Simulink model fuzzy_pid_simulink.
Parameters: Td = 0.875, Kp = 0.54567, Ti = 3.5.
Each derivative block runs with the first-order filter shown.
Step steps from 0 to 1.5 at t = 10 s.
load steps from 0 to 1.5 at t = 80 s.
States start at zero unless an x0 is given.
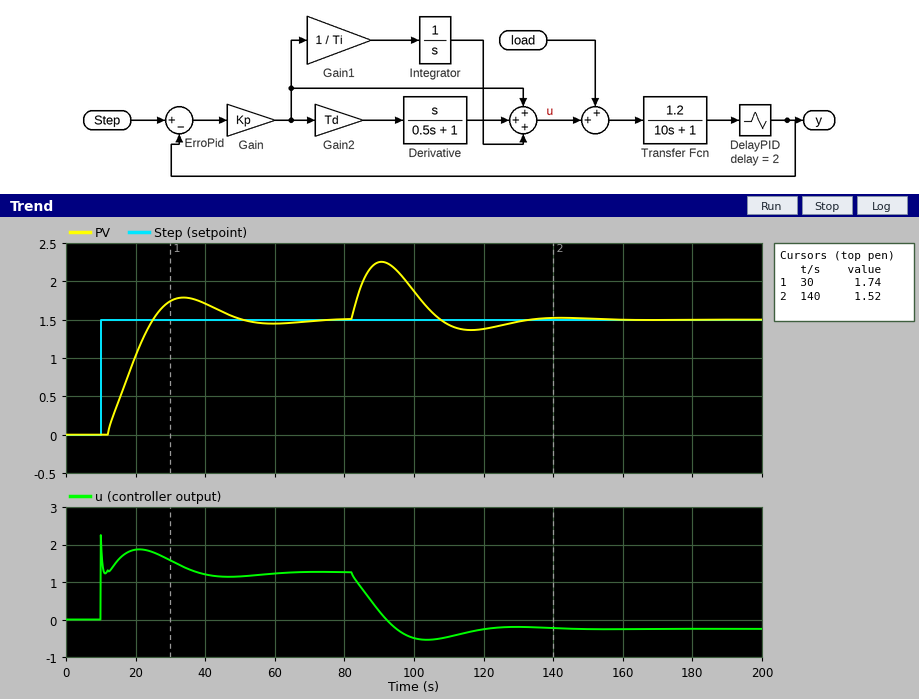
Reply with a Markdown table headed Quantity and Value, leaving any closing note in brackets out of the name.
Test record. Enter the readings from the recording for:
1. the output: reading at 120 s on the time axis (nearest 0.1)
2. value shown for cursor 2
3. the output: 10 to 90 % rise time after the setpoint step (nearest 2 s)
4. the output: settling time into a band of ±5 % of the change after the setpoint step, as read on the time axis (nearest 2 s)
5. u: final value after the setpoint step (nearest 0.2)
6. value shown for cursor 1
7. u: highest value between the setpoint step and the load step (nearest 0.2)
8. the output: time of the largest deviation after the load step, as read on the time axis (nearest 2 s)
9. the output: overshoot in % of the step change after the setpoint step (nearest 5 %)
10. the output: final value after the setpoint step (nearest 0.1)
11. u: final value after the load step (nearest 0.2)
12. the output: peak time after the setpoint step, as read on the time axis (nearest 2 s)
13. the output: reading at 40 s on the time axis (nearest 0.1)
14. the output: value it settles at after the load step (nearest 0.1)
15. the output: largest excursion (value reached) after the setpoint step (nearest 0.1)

| Quantity | Value |
|---|---|
| the output: reading at 120 s on the time axis | 1.4 |
| value shown for cursor 2 | 1.52 |
| the output: 10 to 90 % rise time after the setpoint step | 10 s |
| the output: settling time into a band of ±5 % of the change after the setpoint step, as read on the time axis | 46 s |
| u: final value after the setpoint step | 1.2 |
| value shown for cursor 1 | 1.74 |
| u: highest value between the setpoint step and the load step | 2.2 |
| the output: time of the largest deviation after the load step, as read on the time axis | 90 s |
| the output: overshoot in % of the step change after the setpoint step | 20 % |
| the output: final value after the setpoint step | 1.5 |
| u: final value after the load step | -0.2 |
| the output: peak time after the setpoint step, as read on the time axis | 34 s |
| the output: reading at 40 s on the time axis | 1.7 |
| the output: value it settles at after the load step | 1.5 |
| the output: largest excursion (value reached) after the setpoint step | 1.8 |
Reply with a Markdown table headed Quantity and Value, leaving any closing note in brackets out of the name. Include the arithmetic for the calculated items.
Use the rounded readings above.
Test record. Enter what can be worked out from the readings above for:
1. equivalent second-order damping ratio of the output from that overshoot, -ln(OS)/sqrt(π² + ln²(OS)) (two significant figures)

| Quantity | Value |
|---|---|
| equivalent second-order damping ratio of the output from that overshoot, -ln(OS)/sqrt(π² + ln²(OS)) | ln(0.2) = -1.609; 1.609 / sqrt(9.870 + 2.590) = 0.46 |
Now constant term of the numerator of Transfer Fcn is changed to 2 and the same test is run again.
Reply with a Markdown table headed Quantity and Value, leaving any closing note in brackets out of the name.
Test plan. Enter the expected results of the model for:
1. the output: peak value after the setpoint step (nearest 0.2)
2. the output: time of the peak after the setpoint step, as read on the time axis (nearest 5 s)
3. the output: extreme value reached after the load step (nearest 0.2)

| Quantity | Value |
|---|---|
| the output: peak value after the setpoint step | 1.8 |
| the output: time of the peak after the setpoint step, as read on the time axis | 25 s |
| the output: extreme value reached after the load step | 2.6 |
